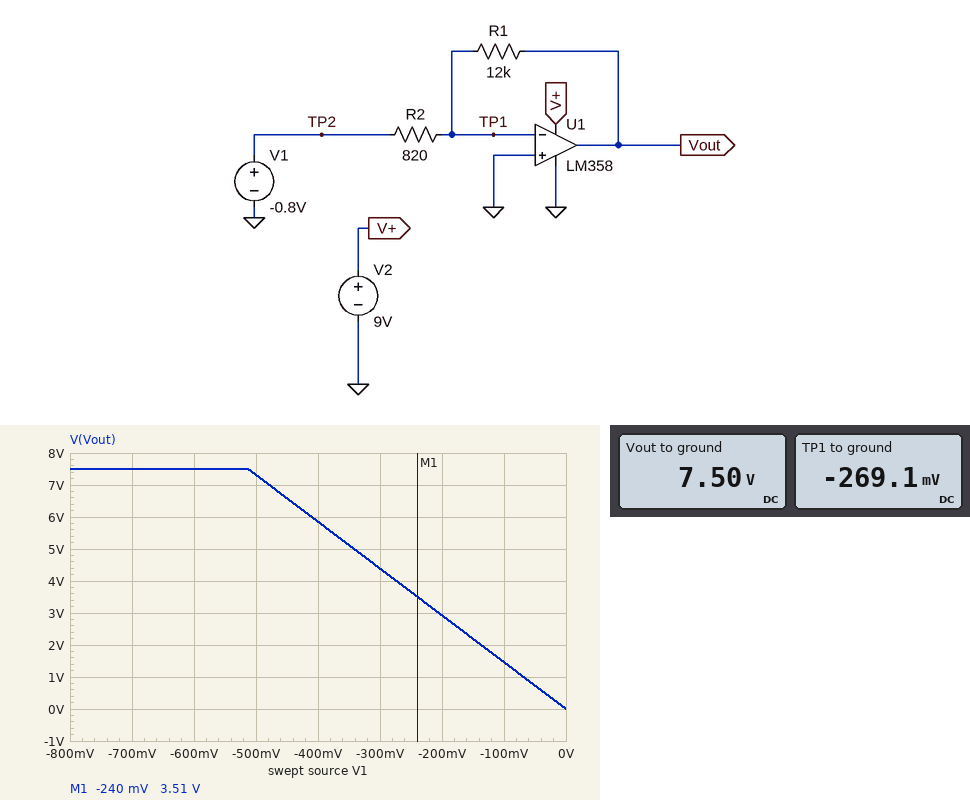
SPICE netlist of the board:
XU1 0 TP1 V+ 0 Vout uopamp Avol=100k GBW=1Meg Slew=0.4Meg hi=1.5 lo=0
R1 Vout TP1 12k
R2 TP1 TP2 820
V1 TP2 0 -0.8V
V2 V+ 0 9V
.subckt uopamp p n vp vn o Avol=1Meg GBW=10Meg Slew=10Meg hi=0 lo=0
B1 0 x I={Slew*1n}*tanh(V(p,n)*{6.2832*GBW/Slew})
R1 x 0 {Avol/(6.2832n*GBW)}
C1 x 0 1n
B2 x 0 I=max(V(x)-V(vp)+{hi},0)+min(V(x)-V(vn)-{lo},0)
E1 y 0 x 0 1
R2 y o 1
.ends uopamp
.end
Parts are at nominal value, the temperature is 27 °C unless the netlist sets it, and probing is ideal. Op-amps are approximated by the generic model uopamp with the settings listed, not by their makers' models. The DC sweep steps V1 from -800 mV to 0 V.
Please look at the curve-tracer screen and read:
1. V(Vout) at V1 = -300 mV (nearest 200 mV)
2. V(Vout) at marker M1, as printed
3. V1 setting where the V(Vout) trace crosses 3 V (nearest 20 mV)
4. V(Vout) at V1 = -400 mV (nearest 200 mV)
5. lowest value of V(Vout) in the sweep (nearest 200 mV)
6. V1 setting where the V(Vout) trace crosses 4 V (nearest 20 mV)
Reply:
4.4 V
3.51 V
-200 mV
5.8 V
0 V
-280 mV
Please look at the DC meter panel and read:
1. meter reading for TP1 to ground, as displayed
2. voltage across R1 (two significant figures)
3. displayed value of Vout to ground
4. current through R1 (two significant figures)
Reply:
-269.1 mV
7.8 V
7.50 V
650 µA
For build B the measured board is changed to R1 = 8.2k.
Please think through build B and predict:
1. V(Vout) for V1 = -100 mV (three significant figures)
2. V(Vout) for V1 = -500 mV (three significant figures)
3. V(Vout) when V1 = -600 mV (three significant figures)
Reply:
1.00 V
5.00 V
6.00 V
